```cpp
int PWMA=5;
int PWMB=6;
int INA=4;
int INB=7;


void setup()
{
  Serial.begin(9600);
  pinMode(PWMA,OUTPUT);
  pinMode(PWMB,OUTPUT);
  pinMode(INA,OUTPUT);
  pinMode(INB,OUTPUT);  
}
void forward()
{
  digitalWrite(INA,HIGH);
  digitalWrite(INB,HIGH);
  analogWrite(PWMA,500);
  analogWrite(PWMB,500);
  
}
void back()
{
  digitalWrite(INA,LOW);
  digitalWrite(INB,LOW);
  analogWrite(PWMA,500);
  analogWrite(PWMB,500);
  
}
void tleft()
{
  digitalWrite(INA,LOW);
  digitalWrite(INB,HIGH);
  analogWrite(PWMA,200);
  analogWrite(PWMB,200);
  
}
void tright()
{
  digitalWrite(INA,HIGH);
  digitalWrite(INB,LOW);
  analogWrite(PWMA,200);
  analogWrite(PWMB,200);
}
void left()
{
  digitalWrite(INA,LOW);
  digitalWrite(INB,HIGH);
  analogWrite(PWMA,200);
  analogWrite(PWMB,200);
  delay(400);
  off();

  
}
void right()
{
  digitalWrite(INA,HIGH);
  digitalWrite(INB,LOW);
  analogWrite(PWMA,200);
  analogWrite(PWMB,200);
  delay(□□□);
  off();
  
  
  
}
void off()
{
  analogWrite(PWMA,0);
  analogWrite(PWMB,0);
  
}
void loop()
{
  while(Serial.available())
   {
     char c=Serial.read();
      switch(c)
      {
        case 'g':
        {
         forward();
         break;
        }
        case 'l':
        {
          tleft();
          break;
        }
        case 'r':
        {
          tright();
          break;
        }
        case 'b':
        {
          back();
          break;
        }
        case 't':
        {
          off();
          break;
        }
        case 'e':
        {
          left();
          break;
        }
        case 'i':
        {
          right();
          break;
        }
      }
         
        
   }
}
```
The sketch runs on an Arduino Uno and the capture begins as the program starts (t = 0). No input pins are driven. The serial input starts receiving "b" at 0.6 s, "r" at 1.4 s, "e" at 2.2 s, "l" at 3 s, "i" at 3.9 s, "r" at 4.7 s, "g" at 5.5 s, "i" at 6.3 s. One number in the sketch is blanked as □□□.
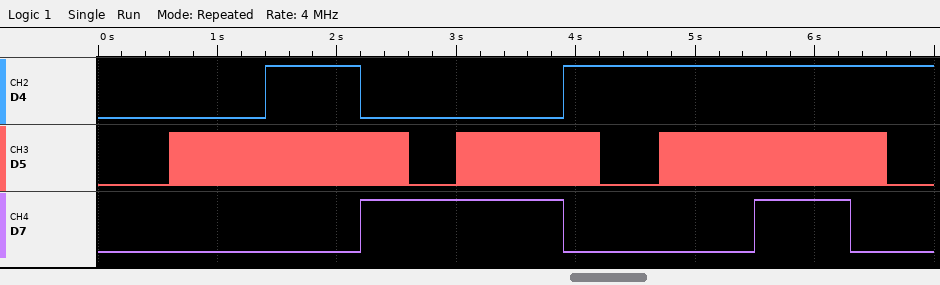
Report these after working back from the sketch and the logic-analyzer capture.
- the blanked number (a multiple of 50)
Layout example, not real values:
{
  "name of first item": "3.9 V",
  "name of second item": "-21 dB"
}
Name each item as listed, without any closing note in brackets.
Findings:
{
  "the blanked number": "300"
}
